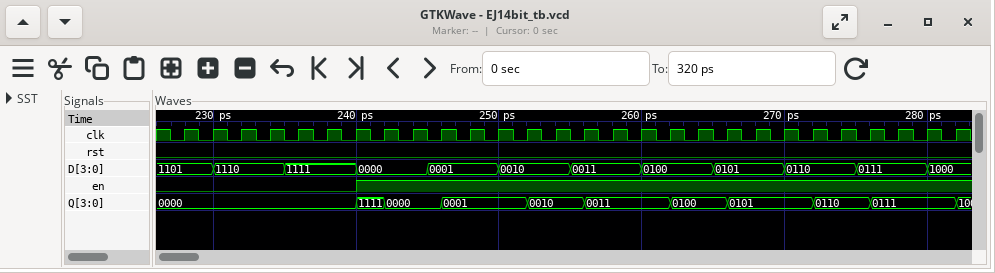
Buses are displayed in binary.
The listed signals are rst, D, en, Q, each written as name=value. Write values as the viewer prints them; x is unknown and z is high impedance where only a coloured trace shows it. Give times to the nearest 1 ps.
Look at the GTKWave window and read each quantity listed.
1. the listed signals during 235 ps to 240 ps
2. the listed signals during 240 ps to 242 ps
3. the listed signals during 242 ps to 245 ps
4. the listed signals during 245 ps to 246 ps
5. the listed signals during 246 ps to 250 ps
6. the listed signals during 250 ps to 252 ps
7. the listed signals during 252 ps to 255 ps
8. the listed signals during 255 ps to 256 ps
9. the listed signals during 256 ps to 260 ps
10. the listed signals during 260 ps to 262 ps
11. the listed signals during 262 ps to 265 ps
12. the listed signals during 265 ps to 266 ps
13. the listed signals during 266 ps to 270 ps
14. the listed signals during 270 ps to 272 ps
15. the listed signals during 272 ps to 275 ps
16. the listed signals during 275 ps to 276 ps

rst=0, D=1111, en=0, Q=0000
rst=0, D=0000, en=1, Q=1111
rst=0, D=0000, en=1, Q=0000
rst=0, D=0001, en=1, Q=0000
rst=0, D=0001, en=1, Q=0001
rst=0, D=0010, en=1, Q=0001
rst=0, D=0010, en=1, Q=0010
rst=0, D=0011, en=1, Q=0010
rst=0, D=0011, en=1, Q=0011
rst=0, D=0100, en=1, Q=0011
rst=0, D=0100, en=1, Q=0100
rst=0, D=0101, en=1, Q=0100
rst=0, D=0101, en=1, Q=0101
rst=0, D=0110, en=1, Q=0101
rst=0, D=0110, en=1, Q=0110
rst=0, D=0111, en=1, Q=0110
